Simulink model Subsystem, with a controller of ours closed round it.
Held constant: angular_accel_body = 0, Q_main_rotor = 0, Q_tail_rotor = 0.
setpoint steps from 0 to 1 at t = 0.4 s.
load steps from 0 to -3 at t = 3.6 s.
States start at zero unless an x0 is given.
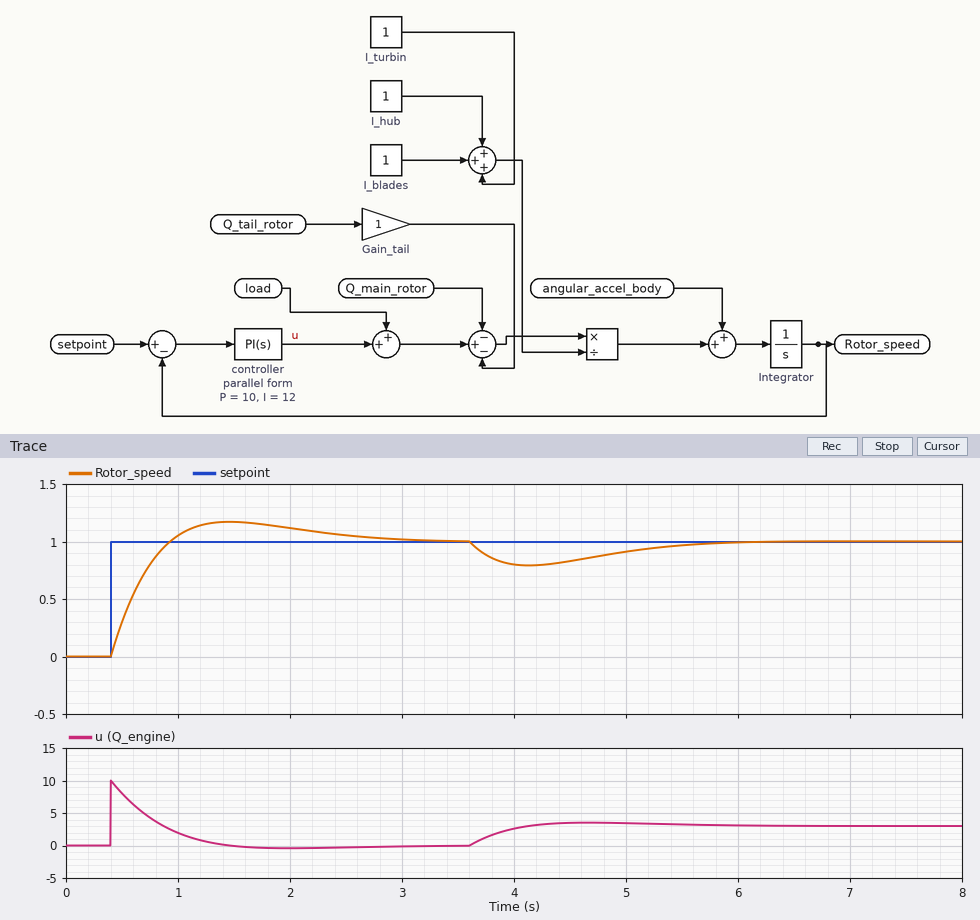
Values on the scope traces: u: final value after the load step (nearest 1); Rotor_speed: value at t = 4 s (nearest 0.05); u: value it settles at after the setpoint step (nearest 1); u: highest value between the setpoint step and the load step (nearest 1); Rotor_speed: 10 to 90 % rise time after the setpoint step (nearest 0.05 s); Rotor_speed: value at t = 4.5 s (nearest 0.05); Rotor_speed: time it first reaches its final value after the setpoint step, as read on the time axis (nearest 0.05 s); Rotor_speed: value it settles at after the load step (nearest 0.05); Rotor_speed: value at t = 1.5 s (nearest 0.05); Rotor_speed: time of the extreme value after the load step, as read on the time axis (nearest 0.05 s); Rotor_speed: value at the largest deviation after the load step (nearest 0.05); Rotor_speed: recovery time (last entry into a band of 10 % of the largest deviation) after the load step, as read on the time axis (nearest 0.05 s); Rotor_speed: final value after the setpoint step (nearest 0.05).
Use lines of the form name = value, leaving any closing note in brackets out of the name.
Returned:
u: final value after the load step = 3
Rotor_speed: value at t = 4 s = 0.80
u: value it settles at after the setpoint step = 0
u: highest value between the setpoint step and the load step = 10
Rotor_speed: 10 to 90 % rise time after the setpoint step = 0.40 s
Rotor_speed: value at t = 4.5 s = 0.85
Rotor_speed: time it first reaches its final value after the setpoint step, as read on the time axis = 0.95 s
Rotor_speed: value it settles at after the load step = 1.00
Rotor_speed: value at t = 1.5 s = 1.15
Rotor_speed: time of the extreme value after the load step, as read on the time axis = 4.15 s
Rotor_speed: value at the largest deviation after the load step = 0.80
Rotor_speed: recovery time (last entry into a band of 10 % of the largest deviation) after the load step, as read on the time axis = 5.70 s
Rotor_speed: final value after the setpoint step = 1.00
